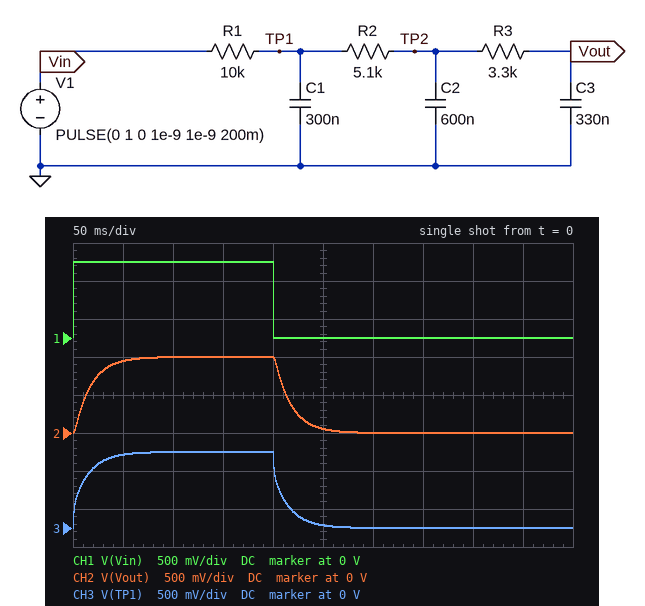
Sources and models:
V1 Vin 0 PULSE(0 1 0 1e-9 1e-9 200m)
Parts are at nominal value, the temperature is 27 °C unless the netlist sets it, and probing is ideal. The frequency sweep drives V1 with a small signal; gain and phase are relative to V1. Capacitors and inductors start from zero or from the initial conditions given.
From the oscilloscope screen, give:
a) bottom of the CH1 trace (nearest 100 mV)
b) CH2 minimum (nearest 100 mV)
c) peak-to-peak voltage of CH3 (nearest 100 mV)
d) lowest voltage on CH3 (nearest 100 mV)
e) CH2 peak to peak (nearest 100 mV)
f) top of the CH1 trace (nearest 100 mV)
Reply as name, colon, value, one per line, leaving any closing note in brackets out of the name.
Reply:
bottom of the CH1 trace: 0 V
CH2 minimum: 0 V
peak-to-peak voltage of CH3: 1.0 V
lowest voltage on CH3: 0 V
CH2 peak to peak: 1.0 V
top of the CH1 trace: 1.0 V
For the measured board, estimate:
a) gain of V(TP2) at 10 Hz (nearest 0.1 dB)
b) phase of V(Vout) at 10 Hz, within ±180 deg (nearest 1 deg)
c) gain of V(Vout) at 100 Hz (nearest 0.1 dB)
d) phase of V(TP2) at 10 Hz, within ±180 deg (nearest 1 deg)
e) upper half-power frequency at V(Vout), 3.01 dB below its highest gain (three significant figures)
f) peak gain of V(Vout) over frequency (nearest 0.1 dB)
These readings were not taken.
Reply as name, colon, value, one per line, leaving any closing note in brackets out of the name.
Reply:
gain of V(TP2) at 10 Hz: -3.2 dB
phase of V(Vout) at 10 Hz, within ±180 deg: -52 deg
gain of V(Vout) at 100 Hz: -22.4 dB
phase of V(TP2) at 10 Hz, within ±180 deg: -48 deg
upper half-power frequency at V(Vout), 3.01 dB below its highest gain: 9.59 Hz
peak gain of V(Vout) over frequency: 0 dB
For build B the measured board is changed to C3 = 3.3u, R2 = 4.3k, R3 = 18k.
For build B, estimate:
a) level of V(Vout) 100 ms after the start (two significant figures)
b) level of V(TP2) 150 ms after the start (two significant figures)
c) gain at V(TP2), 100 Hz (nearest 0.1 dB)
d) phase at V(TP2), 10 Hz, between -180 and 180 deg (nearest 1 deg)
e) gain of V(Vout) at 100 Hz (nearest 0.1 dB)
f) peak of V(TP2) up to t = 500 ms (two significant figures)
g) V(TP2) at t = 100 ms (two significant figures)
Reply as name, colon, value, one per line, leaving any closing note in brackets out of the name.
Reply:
level of V(Vout) 100 ms after the start: 570 mV
level of V(TP2) 150 ms after the start: 870 mV
gain at V(TP2), 100 Hz: -17.9 dB
phase at V(TP2), 10 Hz, between -180 and 180 deg: -30 deg
gain of V(Vout) at 100 Hz: -49.3 dB
peak of V(TP2) up to t = 500 ms: 920 mV
V(TP2) at t = 100 ms: 800 mV
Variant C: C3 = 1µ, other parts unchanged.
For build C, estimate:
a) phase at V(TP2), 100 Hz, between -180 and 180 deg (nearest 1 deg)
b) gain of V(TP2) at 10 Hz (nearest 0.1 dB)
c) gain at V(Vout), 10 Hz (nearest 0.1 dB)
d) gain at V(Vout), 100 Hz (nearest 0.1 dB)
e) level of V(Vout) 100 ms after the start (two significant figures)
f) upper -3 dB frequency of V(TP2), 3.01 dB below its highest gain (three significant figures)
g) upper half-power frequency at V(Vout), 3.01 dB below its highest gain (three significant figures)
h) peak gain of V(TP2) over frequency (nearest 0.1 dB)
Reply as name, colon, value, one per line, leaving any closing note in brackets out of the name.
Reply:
phase at V(TP2), 100 Hz, between -180 and 180 deg: -90 deg
gain of V(TP2) at 10 Hz: -6.0 dB
gain at V(Vout), 10 Hz: -6.2 dB
gain at V(Vout), 100 Hz: -28.6 dB
level of V(Vout) 100 ms after the start: 970 mV
upper -3 dB frequency of V(TP2), 3.01 dB below its highest gain: 5.70 Hz
upper half-power frequency at V(Vout), 3.01 dB below its highest gain: 5.62 Hz
peak gain of V(TP2) over frequency: 0 dB
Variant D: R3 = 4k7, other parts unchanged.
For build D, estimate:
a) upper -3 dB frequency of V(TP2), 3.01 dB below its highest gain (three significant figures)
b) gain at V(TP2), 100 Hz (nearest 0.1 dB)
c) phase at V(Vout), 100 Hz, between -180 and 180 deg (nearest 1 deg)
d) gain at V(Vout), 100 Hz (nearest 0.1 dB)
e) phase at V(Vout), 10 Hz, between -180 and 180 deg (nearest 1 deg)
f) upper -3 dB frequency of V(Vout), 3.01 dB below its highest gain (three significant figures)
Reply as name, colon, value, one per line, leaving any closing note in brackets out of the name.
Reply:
upper -3 dB frequency of V(TP2), 3.01 dB below its highest gain: 9.56 Hz
gain at V(TP2), 100 Hz: -20.3 dB
phase at V(Vout), 100 Hz, between -180 and 180 deg: -146 deg
gain at V(Vout), 100 Hz: -23.2 dB
phase at V(Vout), 10 Hz, between -180 and 180 deg: -53 deg
upper -3 dB frequency of V(Vout), 3.01 dB below its highest gain: 9.48 Hz
